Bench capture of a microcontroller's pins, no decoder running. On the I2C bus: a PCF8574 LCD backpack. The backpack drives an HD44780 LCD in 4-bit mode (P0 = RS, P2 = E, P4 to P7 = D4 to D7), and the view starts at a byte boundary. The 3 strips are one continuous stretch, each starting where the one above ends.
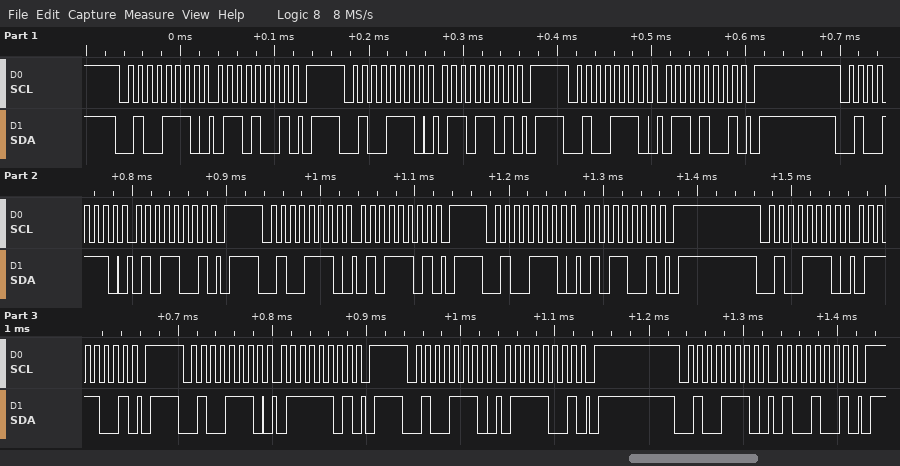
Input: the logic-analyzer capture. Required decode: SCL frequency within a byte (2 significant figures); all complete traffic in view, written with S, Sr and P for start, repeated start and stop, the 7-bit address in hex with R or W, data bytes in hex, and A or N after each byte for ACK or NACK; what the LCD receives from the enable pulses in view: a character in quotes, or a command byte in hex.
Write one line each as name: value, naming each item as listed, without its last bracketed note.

SCL frequency within a byte: 100 kHz
all complete traffic in view, written with S, Sr and P for start, repeated start and stop, the 7-bit address in hex with R or W, data bytes in hex, and A or N after each byte for ACK or NACK: S 27W A 69 A P S 27W A 6D A P S 27W A 69 A P S 27W A 59 A P S 27W A 5D A P S 27W A 59 A P S 27W A 79 A P S 27W A 7D A P S 27W A 79 A P S 27W A 49 A P
what the LCD receives from the enable pulses in view: a character in quotes, or a command byte in hex: 'e'
